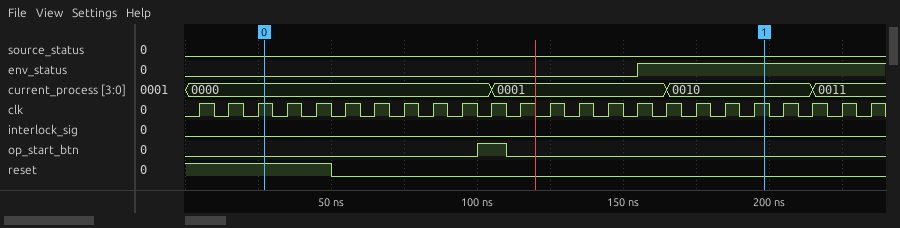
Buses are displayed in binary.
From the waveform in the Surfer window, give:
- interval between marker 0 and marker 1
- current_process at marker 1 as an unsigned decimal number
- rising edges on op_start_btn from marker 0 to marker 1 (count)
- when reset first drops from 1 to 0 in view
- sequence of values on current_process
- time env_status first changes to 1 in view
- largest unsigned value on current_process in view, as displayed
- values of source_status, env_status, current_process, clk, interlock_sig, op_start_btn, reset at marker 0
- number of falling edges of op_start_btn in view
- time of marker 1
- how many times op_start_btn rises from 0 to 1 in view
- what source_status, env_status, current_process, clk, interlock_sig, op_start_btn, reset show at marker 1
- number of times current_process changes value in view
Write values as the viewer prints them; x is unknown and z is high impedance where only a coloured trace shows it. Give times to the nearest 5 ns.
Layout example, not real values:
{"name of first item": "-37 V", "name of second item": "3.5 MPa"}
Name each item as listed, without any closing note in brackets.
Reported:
{"interval between marker 0 and marker 1": "170 ns", "current_process at marker 1 as an unsigned decimal number": "2", "rising edges on op_start_btn from marker 0 to marker 1": "1", "when reset first drops from 1 to 0 in view": "50 ns", "sequence of values on current_process": "0000, 0001, 0010, 0011", "time env_status first changes to 1 in view": "155 ns", "largest unsigned value on current_process in view, as displayed": "0011", "values of source_status, env_status, current_process, clk, interlock_sig, op_start_btn, reset at marker 0": "source_status=0, env_status=0, current_process=0000, clk=1, interlock_sig=0, op_start_btn=0, reset=1", "number of falling edges of op_start_btn in view": "1", "time of marker 1": "200 ns", "how many times op_start_btn rises from 0 to 1 in view": "1", "what source_status, env_status, current_process, clk, interlock_sig, op_start_btn, reset show at marker 1": "source_status=0, env_status=1, current_process=0010, clk=1, interlock_sig=0, op_start_btn=0, reset=0", "number of times current_process changes value in view": "3"}
